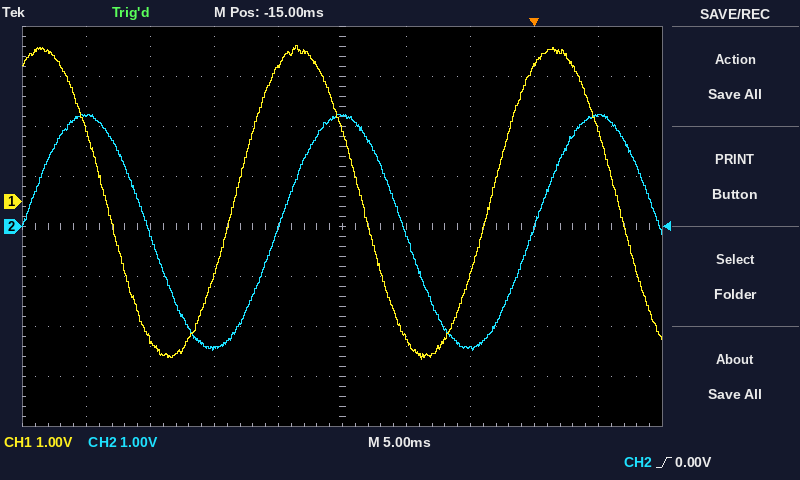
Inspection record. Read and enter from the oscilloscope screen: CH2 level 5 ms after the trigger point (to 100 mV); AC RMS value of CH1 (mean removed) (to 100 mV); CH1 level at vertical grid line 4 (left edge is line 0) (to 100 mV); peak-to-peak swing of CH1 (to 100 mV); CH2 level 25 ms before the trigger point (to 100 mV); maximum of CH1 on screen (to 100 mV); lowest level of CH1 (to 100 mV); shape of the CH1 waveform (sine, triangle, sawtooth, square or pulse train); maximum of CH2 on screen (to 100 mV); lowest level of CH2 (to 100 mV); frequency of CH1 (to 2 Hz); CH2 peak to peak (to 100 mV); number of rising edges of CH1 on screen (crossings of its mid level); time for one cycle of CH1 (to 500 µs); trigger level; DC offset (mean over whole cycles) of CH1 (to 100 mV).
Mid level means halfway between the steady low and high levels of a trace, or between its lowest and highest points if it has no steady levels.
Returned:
2.2 V
2.2 V
2.7 V
6.3 V
-2.4 V
3.1 V
-3.2 V
sine
2.2 V
-2.5 V
50 Hz
4.7 V
2
20.0 ms
0.00 V
0.0 V
